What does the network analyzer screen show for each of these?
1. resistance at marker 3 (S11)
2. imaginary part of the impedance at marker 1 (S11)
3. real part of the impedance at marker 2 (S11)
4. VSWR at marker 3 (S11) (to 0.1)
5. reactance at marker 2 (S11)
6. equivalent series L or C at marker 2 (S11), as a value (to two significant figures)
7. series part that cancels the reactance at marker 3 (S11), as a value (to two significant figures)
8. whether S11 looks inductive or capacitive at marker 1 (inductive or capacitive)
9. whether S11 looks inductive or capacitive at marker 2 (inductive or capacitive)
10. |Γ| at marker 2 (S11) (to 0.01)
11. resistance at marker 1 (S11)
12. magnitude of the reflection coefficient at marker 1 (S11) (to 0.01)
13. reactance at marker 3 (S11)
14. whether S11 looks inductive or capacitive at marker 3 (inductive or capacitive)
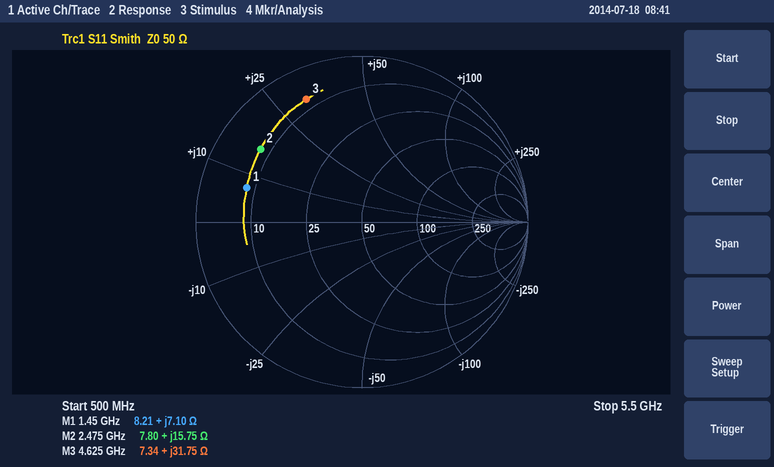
7.34 Ω
+7.10 Ω
7.80 Ω
9.6
+15.75 Ω
1.0 nH
1.1 pF
inductive
inductive
0.75
8.21 Ω
0.72
+31.75 Ω
inductive
